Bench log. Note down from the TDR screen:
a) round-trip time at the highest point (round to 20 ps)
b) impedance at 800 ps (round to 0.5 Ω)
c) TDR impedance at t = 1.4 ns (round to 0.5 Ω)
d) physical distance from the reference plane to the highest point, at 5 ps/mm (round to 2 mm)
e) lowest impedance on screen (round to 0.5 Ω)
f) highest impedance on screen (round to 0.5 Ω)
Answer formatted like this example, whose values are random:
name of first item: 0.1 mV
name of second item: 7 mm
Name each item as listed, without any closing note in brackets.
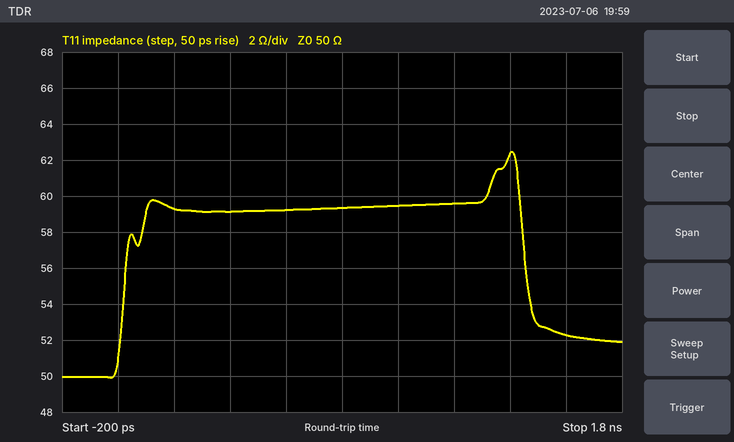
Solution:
round-trip time at the highest point: 1.40 ns
impedance at 800 ps: 59.5 Ω
TDR impedance at t = 1.4 ns: 62.5 Ω
physical distance from the reference plane to the highest point, at 5 ps/mm: 140 mm
lowest impedance on screen: 50.0 Ω
highest impedance on screen: 62.5 Ω
